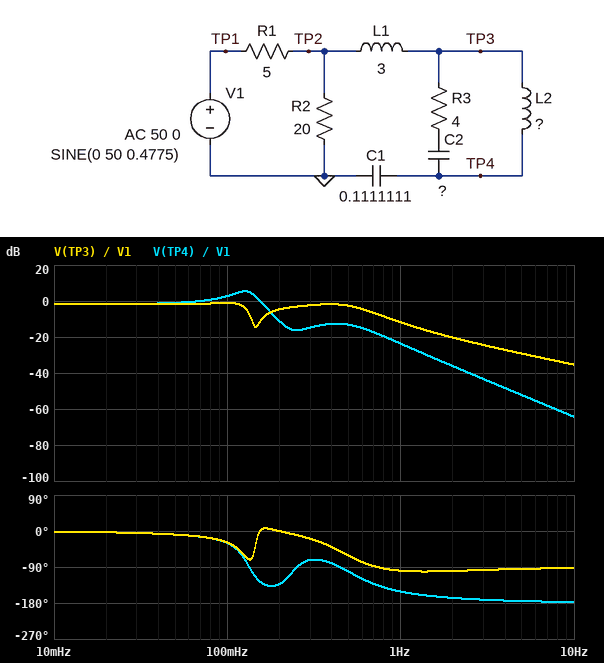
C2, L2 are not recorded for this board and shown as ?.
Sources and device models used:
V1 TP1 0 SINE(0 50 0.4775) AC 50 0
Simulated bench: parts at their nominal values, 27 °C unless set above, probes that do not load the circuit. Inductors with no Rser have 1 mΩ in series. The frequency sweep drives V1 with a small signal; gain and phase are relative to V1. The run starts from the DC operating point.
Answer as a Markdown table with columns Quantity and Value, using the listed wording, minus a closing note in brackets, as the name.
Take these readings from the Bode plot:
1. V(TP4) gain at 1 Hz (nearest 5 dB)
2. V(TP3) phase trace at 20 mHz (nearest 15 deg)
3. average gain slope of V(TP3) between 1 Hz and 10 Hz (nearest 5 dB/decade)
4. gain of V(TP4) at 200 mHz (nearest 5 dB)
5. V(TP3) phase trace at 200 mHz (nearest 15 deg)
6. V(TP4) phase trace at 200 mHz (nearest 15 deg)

| Quantity | Value |
|---|---|
| V(TP4) gain at 1 Hz | -25 dB |
| V(TP3) phase trace at 20 mHz | 0 deg |
| average gain slope of V(TP3) between 1 Hz and 10 Hz | -25 dB/decade |
| gain of V(TP4) at 200 mHz | -10 dB |
| V(TP3) phase trace at 200 mHz | 0 deg |
| V(TP4) phase trace at 200 mHz | -135 deg |
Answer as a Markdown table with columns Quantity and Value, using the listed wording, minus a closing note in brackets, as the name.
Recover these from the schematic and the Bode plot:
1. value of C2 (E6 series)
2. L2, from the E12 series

| Quantity | Value |
|---|---|
| value of C2 | 68 mF |
| L2, from the E12 series | 6.8 H |
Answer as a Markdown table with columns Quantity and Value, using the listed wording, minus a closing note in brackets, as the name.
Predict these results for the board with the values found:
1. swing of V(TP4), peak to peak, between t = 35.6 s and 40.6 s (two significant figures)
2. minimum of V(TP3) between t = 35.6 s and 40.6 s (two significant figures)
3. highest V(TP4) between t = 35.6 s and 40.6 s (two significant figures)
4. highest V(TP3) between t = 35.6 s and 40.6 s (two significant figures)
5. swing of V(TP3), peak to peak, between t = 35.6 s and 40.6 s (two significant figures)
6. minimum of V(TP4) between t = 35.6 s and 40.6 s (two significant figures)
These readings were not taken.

| Quantity | Value |
|---|---|
| swing of V(TP4), peak to peak, between t = 35.6 s and 40.6 s | 23 V |
| minimum of V(TP3) between t = 35.6 s and 40.6 s | -38 V |
| highest V(TP4) between t = 35.6 s and 40.6 s | 11 V |
| highest V(TP3) between t = 35.6 s and 40.6 s | 38 V |
| swing of V(TP3), peak to peak, between t = 35.6 s and 40.6 s | 77 V |
| minimum of V(TP4) between t = 35.6 s and 40.6 s | -11 V |
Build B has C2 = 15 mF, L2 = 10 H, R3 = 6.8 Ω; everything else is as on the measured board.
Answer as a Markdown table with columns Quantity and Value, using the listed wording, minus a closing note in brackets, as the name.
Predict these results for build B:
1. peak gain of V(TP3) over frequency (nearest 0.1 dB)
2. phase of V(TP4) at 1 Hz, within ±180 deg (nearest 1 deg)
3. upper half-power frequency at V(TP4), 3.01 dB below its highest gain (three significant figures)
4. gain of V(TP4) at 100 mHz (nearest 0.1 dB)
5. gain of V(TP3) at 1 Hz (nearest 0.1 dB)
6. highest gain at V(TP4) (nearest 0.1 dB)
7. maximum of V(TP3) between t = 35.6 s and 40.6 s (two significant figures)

| Quantity | Value |
|---|---|
| peak gain of V(TP3) over frequency | 0.4 dB |
| phase of V(TP4) at 1 Hz, within ±180 deg | -113 deg |
| upper half-power frequency at V(TP4), 3.01 dB below its highest gain | 143 mHz |
| gain of V(TP4) at 100 mHz | 4.2 dB |
| gain of V(TP3) at 1 Hz | -1.2 dB |
| highest gain at V(TP4) | 7.0 dB |
| maximum of V(TP3) between t = 35.6 s and 40.6 s | 41 V |
